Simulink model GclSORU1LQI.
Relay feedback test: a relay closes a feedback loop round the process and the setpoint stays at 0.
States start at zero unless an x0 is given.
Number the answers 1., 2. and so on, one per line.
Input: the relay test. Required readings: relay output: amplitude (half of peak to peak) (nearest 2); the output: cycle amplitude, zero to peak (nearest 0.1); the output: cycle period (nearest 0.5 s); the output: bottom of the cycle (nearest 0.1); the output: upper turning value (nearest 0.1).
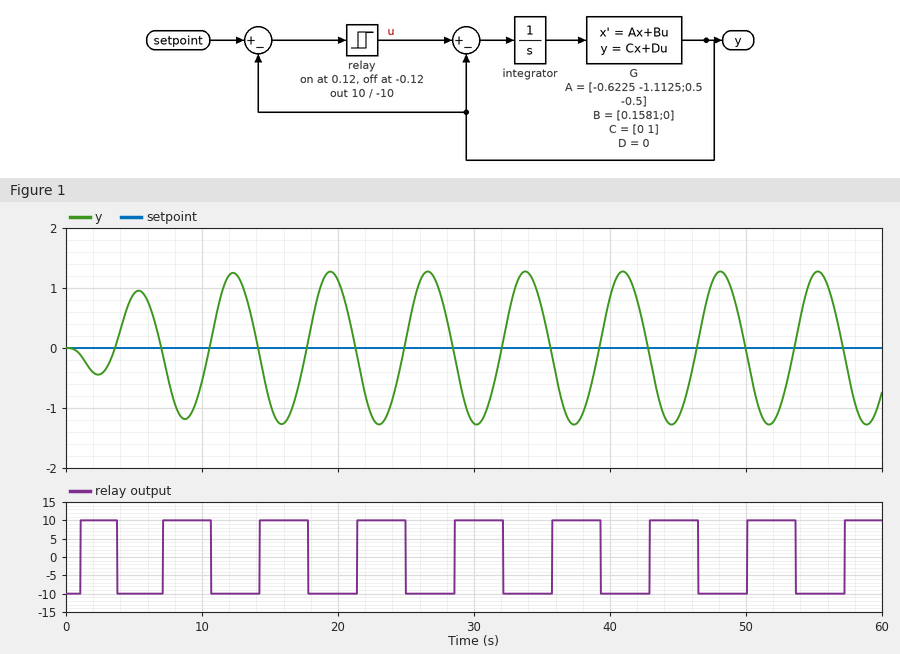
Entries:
1. 10
2. 1.3
3. 7.0 s
4. -1.3
5. 1.3
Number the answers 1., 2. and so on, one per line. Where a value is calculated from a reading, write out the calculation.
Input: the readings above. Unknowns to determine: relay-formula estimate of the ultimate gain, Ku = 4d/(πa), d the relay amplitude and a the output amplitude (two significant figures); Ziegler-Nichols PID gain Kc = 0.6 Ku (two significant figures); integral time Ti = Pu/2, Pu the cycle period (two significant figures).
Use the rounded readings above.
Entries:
1. 4 × 10 / (π × 1.3) = 9.8
2. 0.6 × 9.8 = 5.9
3. 7 / 2 = 3.5 s
